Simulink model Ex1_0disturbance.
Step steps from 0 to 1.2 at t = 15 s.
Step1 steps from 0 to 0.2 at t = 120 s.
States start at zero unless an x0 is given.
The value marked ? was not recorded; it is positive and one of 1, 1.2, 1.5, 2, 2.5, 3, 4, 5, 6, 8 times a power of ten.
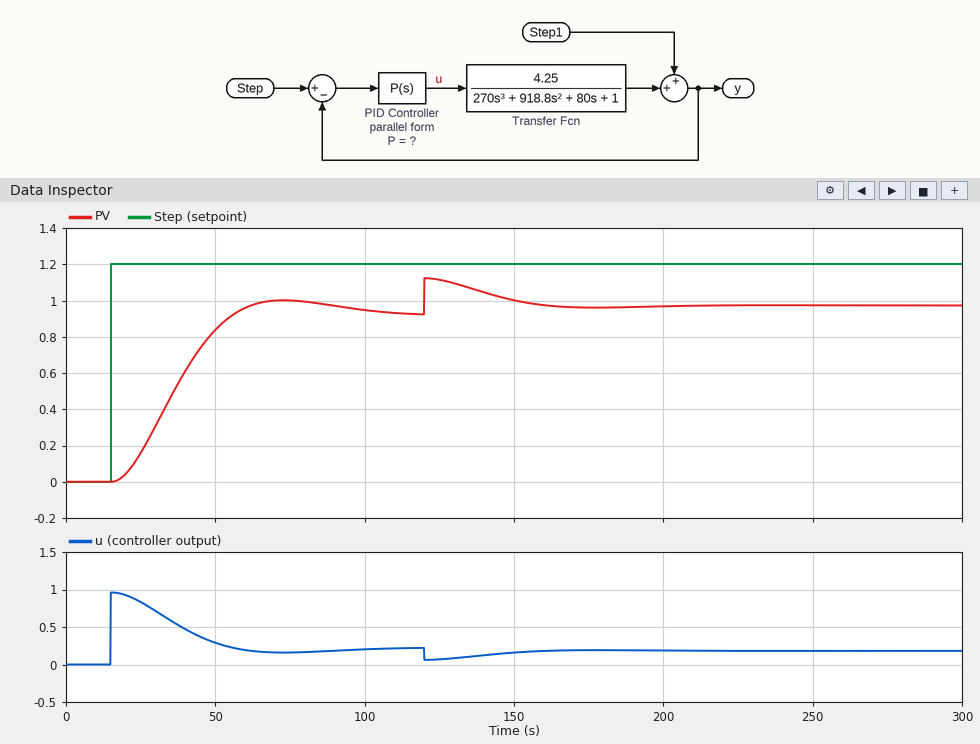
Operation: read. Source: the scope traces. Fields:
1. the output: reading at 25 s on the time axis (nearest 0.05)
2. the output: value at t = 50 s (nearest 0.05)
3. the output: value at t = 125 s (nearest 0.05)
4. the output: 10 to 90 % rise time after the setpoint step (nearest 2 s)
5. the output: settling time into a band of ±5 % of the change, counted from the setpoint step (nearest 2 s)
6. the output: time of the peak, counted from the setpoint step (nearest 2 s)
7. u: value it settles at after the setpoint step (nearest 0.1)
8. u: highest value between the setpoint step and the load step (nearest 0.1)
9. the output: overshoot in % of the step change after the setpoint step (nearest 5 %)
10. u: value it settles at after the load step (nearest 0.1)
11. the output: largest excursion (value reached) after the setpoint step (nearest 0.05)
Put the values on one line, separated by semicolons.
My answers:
0.15; 0.85; 1.10; 28 s; 74 s; 58 s; 0.2; 1.0; 10 %; 0.2; 1.00
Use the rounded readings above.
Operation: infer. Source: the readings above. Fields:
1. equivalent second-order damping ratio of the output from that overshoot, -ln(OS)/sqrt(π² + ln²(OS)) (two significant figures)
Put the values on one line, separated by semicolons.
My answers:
0.59
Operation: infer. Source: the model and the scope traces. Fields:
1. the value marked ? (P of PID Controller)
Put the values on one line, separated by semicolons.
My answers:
0.8
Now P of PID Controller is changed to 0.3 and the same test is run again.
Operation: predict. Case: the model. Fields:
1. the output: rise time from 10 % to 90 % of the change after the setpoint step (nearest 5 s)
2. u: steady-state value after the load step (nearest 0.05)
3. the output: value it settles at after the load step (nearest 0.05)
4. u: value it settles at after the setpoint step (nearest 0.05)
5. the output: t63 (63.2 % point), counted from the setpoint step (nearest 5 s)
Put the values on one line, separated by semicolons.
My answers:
55 s; 0.15; 0.75; 0.15; 40 s
